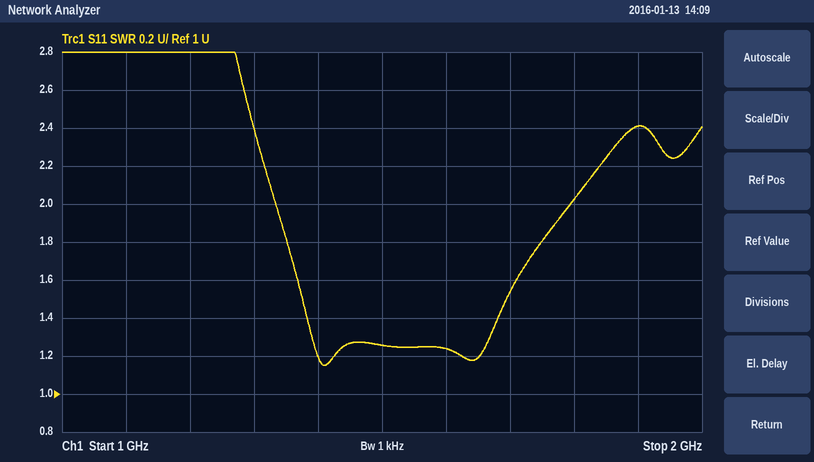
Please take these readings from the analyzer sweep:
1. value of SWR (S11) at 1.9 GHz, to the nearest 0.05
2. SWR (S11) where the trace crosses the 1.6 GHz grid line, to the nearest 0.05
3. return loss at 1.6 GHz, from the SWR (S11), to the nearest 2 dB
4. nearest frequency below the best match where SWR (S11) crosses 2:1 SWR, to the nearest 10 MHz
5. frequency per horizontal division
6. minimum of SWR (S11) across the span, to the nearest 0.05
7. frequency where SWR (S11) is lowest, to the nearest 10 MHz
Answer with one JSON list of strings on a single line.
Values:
["2.40", "1.25", "20 dB", "1.33 GHz", "100 MHz", "1.15", "1.41 GHz"]
